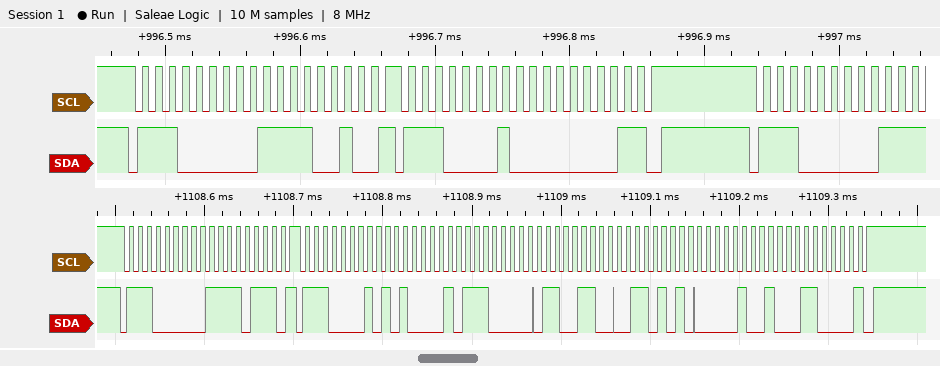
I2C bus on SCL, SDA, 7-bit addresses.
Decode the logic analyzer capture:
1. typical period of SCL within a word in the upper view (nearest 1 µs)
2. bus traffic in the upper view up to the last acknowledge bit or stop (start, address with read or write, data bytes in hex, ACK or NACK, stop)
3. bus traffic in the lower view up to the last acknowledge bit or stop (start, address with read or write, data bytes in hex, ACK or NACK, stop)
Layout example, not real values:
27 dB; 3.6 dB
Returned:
10 µs; start, address 70 write ACK, F2 ACK, repeated start, address 70 read ACK, 01 NACK, stop, start, address 70 write ACK; start, address 70 write ACK, F7 ACK, repeated start, address 70 read ACK, A1 ACK, E0 ACK, CC ACK, 6A ACK, 09 ACK, 30 NACK, stop
